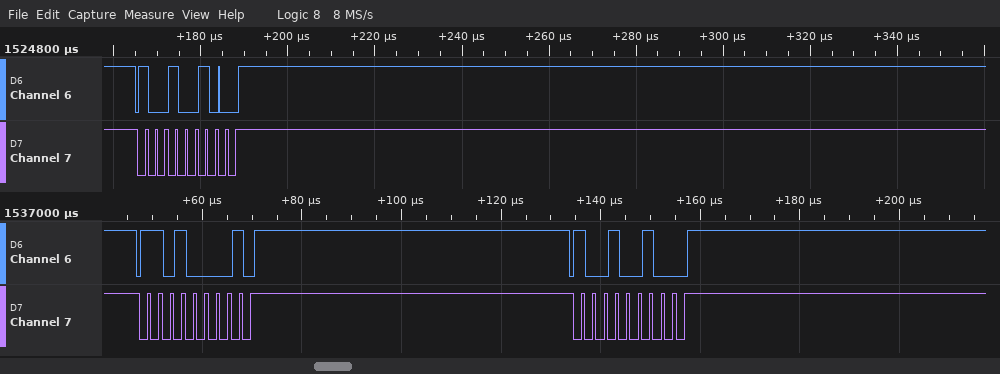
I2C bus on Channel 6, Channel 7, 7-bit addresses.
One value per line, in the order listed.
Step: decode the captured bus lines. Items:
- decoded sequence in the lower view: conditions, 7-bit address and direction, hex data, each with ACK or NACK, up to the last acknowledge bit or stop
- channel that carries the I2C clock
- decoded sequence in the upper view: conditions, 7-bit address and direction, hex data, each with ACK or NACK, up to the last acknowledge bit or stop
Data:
start, address 68 write NACK, stop, start, address 49 write ACK, stop
Channel 7
start, address 49 write ACK, stop
